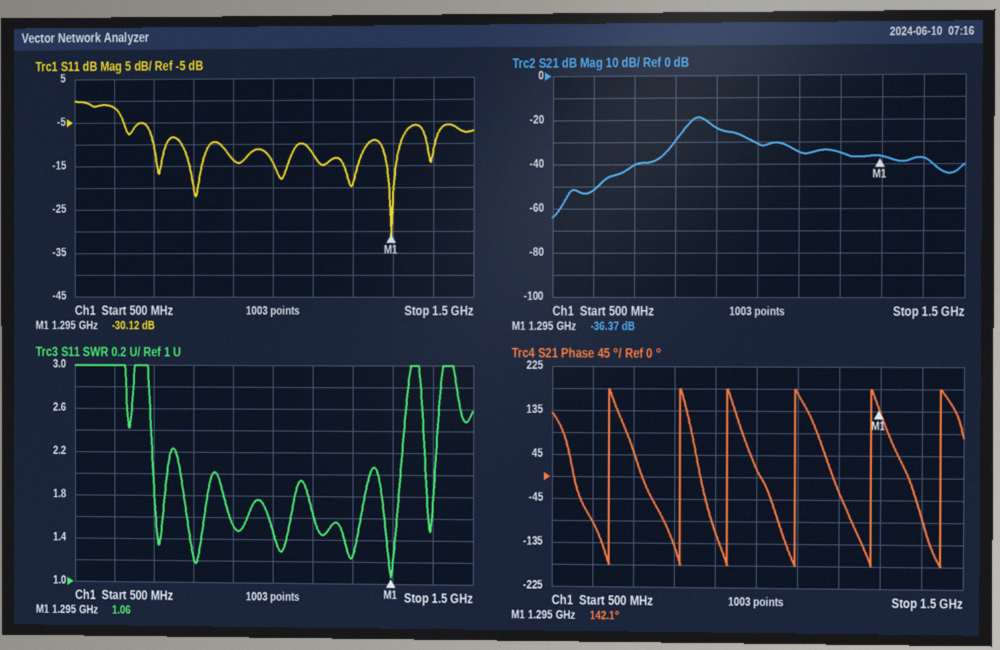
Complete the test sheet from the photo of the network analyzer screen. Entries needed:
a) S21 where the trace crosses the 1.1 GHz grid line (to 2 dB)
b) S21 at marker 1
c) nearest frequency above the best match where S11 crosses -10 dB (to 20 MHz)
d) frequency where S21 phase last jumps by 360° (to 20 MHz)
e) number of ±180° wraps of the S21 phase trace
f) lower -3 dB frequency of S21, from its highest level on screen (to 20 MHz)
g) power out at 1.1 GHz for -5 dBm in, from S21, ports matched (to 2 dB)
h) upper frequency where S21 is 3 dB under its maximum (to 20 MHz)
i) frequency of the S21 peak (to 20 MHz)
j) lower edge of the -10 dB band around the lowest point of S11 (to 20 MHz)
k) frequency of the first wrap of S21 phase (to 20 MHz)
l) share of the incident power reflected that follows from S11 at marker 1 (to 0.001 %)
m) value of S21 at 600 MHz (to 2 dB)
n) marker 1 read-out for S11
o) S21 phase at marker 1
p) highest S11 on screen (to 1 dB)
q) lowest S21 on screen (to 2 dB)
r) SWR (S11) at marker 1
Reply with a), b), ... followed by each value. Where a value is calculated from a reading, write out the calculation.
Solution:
a) -34 dB
b) -36.37 dB
c) 1.32 GHz
d) 1.44 GHz
e) 6
f) 840 MHz
g) -5 dBm + (-34 dB) = -40 dBm
h) 880 MHz
i) 860 MHz
j) 1.26 GHz
k) 640 MHz
l) 10^(-30.12/10) ≈ 0.097 %
m) -52 dB
n) -30.12 dB
o) 142.1°
p) 0 dB
q) -64 dB
r) 1.06
